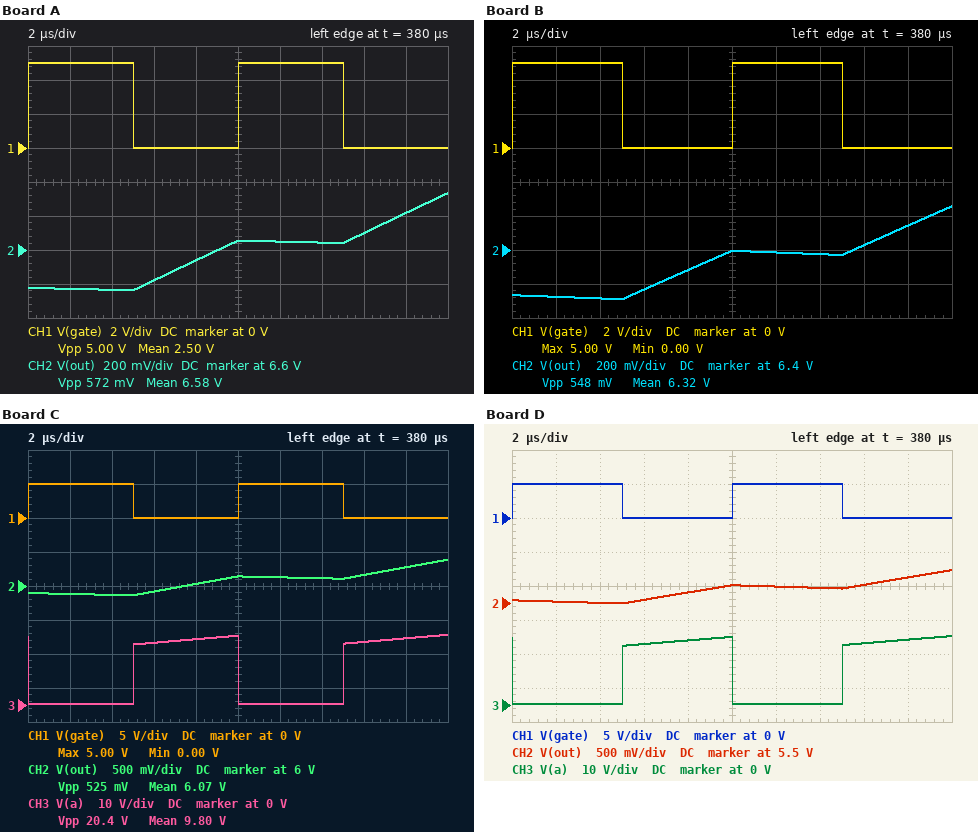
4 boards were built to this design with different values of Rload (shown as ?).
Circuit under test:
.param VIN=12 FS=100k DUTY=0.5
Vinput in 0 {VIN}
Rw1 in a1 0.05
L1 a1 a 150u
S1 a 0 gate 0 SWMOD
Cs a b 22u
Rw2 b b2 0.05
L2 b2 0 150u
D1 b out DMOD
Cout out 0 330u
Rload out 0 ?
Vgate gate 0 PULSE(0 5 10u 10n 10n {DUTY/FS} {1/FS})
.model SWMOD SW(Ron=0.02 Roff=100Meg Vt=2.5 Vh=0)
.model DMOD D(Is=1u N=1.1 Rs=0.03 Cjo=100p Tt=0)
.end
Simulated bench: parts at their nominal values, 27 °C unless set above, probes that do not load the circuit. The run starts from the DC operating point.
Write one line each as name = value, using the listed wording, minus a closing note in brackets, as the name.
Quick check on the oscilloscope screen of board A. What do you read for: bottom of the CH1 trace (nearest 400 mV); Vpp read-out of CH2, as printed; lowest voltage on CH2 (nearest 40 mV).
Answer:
bottom of the CH1 trace = 0 V
Vpp read-out of CH2, as printed = 572 mV
lowest voltage on CH2 = 6.36 V
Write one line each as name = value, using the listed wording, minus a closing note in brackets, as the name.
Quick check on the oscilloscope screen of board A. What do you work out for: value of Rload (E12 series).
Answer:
value of Rload = 6.8 Ω
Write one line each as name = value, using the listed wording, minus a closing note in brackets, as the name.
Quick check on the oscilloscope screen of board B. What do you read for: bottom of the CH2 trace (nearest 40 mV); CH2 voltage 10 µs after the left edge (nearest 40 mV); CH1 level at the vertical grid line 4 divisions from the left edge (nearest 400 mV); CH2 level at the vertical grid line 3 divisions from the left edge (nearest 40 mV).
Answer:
bottom of the CH2 trace = 6.12 V
CH2 voltage 10 µs after the left edge = 6.40 V
CH1 level at the vertical grid line 4 divisions from the left edge = 0 V
CH2 level at the vertical grid line 3 divisions from the left edge = 6.16 V
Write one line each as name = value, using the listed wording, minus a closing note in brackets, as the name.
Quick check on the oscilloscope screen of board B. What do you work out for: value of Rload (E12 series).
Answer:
value of Rload = 3.9 Ω
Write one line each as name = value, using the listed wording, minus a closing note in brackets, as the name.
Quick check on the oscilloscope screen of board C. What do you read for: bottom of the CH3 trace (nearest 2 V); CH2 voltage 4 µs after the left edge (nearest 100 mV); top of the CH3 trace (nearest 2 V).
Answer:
bottom of the CH3 trace = 0 V
CH2 voltage 4 µs after the left edge = 5.9 V
top of the CH3 trace = 20 V
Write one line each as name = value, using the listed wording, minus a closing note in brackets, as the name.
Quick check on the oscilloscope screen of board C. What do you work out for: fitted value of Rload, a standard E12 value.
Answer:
fitted value of Rload, a standard E12 value = 2.7 Ω
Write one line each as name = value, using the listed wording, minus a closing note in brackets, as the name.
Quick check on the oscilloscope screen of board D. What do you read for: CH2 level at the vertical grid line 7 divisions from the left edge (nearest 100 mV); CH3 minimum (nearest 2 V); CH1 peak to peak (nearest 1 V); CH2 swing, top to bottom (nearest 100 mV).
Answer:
CH2 level at the vertical grid line 7 divisions from the left edge = 5.7 V
CH3 minimum = 0 V
CH1 peak to peak = 5 V
CH2 swing, top to bottom = 500 mV
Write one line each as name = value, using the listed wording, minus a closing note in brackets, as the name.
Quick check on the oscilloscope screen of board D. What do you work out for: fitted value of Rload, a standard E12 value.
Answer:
fitted value of Rload, a standard E12 value = 1.8 Ω
